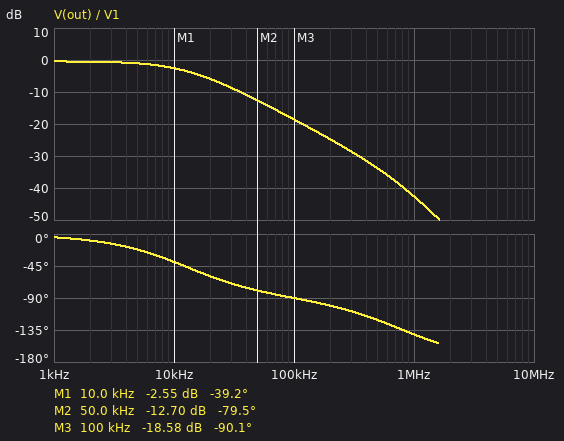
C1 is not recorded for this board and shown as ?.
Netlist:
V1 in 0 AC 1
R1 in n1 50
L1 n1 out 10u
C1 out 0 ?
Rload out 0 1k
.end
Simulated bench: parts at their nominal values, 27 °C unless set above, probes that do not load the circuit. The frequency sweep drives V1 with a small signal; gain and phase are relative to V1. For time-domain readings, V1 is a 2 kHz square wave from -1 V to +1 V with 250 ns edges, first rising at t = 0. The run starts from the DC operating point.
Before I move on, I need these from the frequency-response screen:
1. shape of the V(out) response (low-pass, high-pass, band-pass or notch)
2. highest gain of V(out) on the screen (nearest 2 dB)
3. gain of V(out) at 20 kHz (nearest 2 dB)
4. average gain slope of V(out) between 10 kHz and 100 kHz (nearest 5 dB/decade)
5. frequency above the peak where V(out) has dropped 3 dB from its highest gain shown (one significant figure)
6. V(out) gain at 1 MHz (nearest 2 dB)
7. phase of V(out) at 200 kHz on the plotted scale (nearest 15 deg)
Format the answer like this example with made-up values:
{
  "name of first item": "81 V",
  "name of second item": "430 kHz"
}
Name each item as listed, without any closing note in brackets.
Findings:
{
  "shape of the V(out) response": "low-pass",
  "highest gain of V(out) on the screen": "0 dB",
  "gain of V(out) at 20 kHz": "-6 dB",
  "average gain slope of V(out) between 10 kHz and 100 kHz": "-15 dB/decade",
  "frequency above the peak where V(out) has dropped 3 dB from its highest gain shown": "10 kHz",
  "V(out) gain at 1 MHz": "-42 dB",
  "phase of V(out) at 200 kHz on the plotted scale": "-105 deg"
}
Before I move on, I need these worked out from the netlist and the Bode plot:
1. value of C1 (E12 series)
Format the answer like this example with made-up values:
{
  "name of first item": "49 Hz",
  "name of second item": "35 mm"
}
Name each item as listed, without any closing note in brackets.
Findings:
{
  "value of C1": "270 nF"
}
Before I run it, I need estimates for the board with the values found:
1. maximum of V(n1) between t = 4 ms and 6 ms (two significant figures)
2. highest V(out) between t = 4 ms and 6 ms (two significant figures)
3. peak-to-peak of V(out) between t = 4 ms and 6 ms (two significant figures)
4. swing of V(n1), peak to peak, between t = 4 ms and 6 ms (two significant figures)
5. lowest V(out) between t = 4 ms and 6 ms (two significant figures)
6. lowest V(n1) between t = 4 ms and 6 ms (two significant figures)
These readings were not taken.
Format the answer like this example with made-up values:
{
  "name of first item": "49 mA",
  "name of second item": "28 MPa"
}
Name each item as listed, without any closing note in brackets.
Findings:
{
  "maximum of V(n1) between t = 4 ms and 6 ms": "950 mV",
  "highest V(out) between t = 4 ms and 6 ms": "950 mV",
  "peak-to-peak of V(out) between t = 4 ms and 6 ms": "1.9 V",
  "swing of V(n1), peak to peak, between t = 4 ms and 6 ms": "1.9 V",
  "lowest V(out) between t = 4 ms and 6 ms": "-950 mV",
  "lowest V(n1) between t = 4 ms and 6 ms": "-950 mV"
}
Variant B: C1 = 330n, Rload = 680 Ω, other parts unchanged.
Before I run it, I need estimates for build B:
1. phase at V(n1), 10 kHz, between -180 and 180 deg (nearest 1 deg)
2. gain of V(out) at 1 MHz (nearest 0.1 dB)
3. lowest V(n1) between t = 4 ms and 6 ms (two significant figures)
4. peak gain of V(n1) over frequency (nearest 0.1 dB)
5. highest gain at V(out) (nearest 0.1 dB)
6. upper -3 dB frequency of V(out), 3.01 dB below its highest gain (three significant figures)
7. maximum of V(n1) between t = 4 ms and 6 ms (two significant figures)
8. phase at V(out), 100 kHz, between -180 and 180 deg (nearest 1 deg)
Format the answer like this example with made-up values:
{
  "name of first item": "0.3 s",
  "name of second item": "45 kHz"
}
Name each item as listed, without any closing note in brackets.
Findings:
{
  "phase at V(n1), 10 kHz, between -180 and 180 deg": "-44 deg",
  "gain of V(out) at 1 MHz": "-44.4 dB",
  "lowest V(n1) between t = 4 ms and 6 ms": "-930 mV",
  "peak gain of V(n1) over frequency": "0 dB",
  "highest gain at V(out)": "-0.6 dB",
  "upper -3 dB frequency of V(out), 3.01 dB below its highest gain": "10.5 kHz",
  "maximum of V(n1) between t = 4 ms and 6 ms": "930 mV",
  "phase at V(out), 100 kHz, between -180 and 180 deg": "-91 deg"
}
